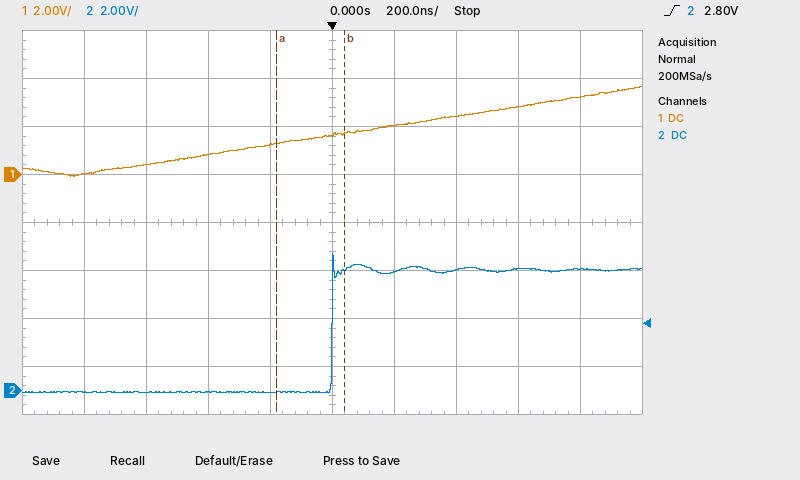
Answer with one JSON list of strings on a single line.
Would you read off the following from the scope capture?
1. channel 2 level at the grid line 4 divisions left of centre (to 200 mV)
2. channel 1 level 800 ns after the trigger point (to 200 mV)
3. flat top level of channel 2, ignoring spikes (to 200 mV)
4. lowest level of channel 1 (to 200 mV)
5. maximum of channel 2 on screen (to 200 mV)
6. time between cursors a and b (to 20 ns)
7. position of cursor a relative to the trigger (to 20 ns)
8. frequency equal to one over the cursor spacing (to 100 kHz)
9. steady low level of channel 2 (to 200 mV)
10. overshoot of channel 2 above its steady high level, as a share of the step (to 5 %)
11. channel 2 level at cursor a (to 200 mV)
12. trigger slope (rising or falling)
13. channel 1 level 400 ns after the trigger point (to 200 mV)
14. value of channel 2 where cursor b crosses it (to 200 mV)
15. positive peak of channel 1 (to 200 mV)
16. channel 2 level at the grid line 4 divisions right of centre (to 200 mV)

["0.0 V", "3.2 V", "5.0 V", "0.0 V", "5.8 V", "220 ns", "-180 ns", "4.5 MHz", "0.0 V", "15 %", "0.0 V", "rising", "2.4 V", "5.0 V", "3.6 V", "5.0 V"]
